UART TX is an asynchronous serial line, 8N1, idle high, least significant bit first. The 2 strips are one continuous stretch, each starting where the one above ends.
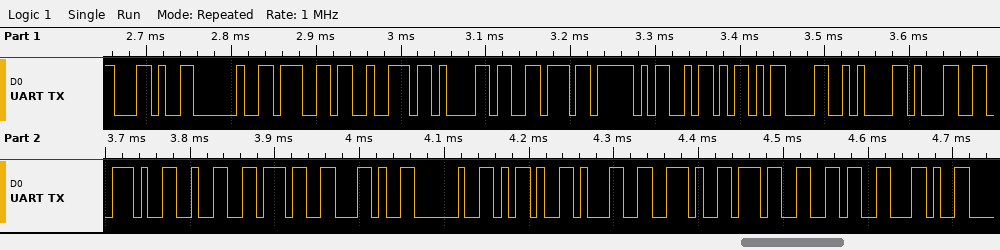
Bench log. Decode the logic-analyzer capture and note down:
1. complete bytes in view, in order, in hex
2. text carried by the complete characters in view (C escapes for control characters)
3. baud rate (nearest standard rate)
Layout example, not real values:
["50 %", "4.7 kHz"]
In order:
["2C 20 67 72 61 76 5F 5A 0D 0A 31 2E 32 37 2C 20 2D 31 2E 37 36 2C", "\", grav_Z\\r\\n1.27, -1.76,\"", "115200 baud"]
